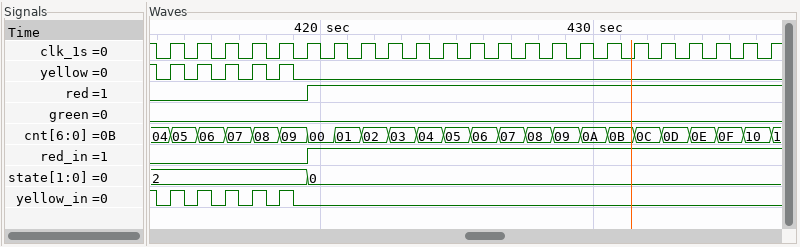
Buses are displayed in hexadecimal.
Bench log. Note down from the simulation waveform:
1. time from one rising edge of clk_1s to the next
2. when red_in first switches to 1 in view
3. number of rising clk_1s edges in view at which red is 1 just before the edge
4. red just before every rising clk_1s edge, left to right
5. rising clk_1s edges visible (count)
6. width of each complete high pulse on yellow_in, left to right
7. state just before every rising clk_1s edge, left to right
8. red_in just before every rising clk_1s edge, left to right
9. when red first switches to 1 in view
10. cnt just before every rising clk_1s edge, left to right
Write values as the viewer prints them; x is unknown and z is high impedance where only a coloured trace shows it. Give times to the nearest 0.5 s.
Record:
1 s
419.5 s
17
0 0 0 0 0 0 1 1 1 1 1 1 1 1 1 1 1 1 1 1 1 1 1
23
0.5 s, 0.5 s, 0.5 s, 0.5 s, 0.5 s
2, 2, 2, 2, 2, 2, 0, 0, 0, 0, 0, 0, 0, 0, 0, 0, 0, 0, 0, 0, 0, 0, 0
0 0 0 0 0 0 1 1 1 1 1 1 1 1 1 1 1 1 1 1 1 1 1
419.5 s
04, 05, 06, 07, 08, 09, 00, 01, 02, 03, 04, 05, 06, 07, 08, 09, 0A, 0B, 0C, 0D, 0E, 0F, 10
